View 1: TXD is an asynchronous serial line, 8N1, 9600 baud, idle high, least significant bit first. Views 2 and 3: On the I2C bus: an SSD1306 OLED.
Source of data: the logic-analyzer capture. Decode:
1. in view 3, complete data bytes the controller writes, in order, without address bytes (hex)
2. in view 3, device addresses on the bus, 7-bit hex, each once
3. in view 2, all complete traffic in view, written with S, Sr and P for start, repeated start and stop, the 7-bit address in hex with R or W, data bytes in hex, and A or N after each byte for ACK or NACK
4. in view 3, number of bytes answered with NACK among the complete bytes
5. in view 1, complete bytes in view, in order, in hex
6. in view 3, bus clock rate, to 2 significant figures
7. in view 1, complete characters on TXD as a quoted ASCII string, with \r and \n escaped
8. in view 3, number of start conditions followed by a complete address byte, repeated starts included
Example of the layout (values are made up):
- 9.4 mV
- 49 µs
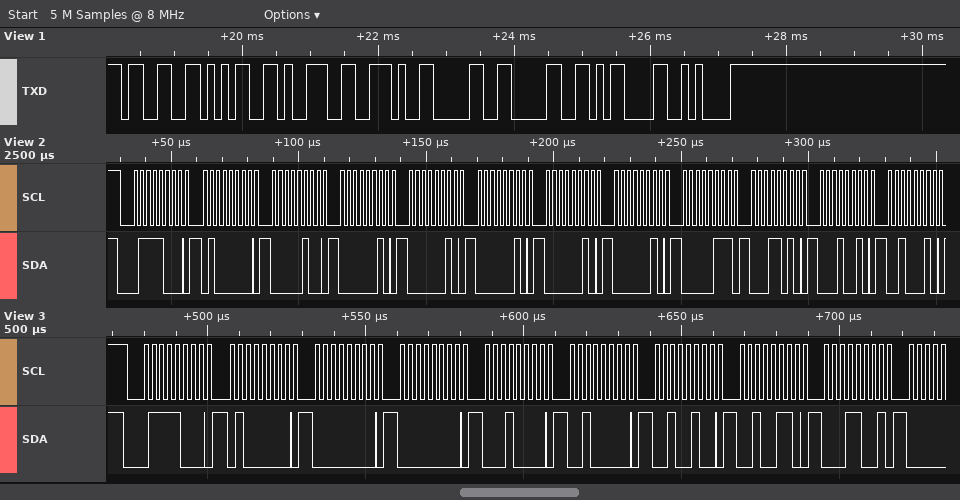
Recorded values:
- 40 00 00 10 20 24 26 19
- 0x3C
- S 3CW A 40 A 04 A 02 A 02 A 02 A 02 A 02 A 07 A 1A A 12 A 22 A
- 0
- 0x33 0x35 0x39 0x2E 0x30 0x30 0x0D 0x0A
- 400 kHz
- "359.00\r\n"
- 1
